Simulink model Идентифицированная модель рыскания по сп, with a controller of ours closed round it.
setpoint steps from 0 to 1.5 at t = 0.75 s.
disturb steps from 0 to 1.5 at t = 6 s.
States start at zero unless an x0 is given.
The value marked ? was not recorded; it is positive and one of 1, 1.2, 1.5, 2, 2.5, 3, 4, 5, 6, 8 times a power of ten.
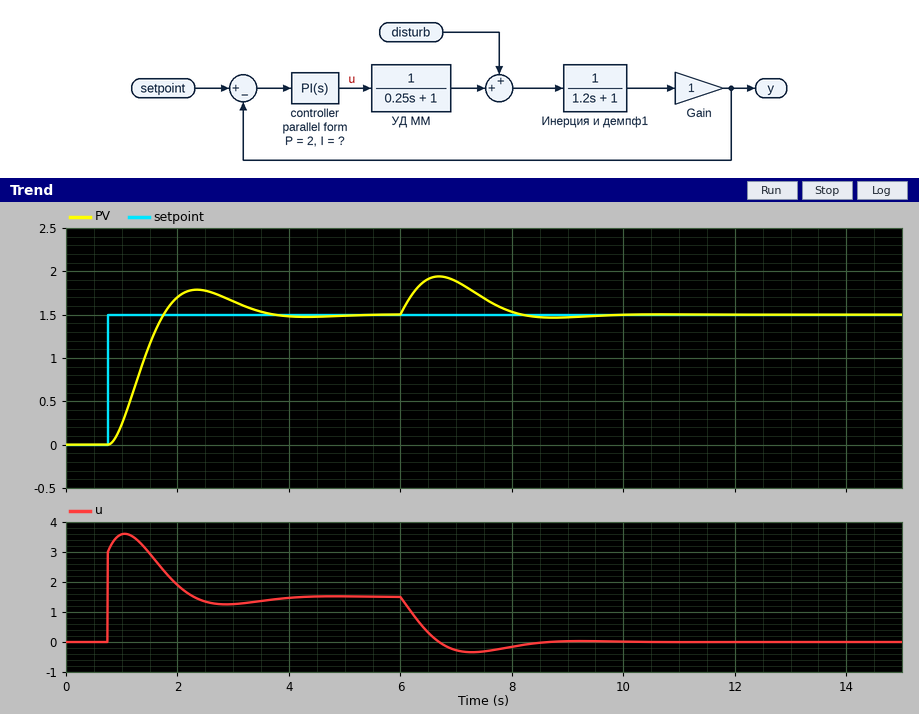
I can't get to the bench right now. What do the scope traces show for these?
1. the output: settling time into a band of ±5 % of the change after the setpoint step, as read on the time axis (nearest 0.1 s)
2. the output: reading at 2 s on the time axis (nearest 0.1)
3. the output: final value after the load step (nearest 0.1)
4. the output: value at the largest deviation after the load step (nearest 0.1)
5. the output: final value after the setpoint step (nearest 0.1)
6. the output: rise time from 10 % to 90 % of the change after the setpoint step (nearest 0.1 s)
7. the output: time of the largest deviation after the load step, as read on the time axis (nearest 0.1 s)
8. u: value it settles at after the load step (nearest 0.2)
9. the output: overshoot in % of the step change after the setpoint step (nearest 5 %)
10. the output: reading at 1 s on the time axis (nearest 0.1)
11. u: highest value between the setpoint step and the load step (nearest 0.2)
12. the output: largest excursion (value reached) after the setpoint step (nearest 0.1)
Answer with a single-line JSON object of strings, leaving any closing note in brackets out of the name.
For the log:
{"the output: settling time into a band of ±5 % of the change after the setpoint step, as read on the time axis": "3.3 s", "the output: reading at 2 s on the time axis": "1.7", "the output: final value after the load step": "1.5", "the output: value at the largest deviation after the load step": "1.9", "the output: final value after the setpoint step": "1.5", "the output: rise time from 10 % to 90 % of the change after the setpoint step": "0.7 s", "the output: time of the largest deviation after the load step, as read on the time axis": "6.7 s", "u: value it settles at after the load step": "0.0", "the output: overshoot in % of the step change after the setpoint step": "20 %", "the output: reading at 1 s on the time axis": "0.2", "u: highest value between the setpoint step and the load step": "3.6", "the output: largest excursion (value reached) after the setpoint step": "1.8"}
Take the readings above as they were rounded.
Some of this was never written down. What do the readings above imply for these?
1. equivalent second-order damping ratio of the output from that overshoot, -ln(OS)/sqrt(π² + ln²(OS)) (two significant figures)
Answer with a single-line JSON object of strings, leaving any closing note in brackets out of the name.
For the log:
{"equivalent second-order damping ratio of the output from that overshoot, -ln(OS)/sqrt(π² + ln²(OS))": "0.46"}
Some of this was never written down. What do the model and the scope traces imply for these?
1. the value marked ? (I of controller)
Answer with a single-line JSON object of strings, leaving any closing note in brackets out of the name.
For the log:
{"the value marked ?": "3"}
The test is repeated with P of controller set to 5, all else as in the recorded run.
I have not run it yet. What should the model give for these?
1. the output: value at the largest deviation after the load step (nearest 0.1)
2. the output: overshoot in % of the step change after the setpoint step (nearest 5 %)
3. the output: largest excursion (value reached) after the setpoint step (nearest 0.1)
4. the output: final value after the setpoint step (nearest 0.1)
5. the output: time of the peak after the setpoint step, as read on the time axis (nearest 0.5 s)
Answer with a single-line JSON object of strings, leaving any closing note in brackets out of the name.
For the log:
{"the output: value at the largest deviation after the load step": "1.8", "the output: overshoot in % of the step change after the setpoint step": "10 %", "the output: largest excursion (value reached) after the setpoint step": "1.7", "the output: final value after the setpoint step": "1.5", "the output: time of the peak after the setpoint step, as read on the time axis": "1.5 s"}
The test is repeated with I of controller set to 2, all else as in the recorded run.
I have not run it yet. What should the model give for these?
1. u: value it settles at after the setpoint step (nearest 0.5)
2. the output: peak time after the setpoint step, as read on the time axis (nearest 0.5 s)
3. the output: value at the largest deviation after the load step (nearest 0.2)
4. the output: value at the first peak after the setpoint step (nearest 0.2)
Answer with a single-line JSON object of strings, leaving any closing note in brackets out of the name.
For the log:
{"u: value it settles at after the setpoint step": "1.5", "the output: peak time after the setpoint step, as read on the time axis": "2.5 s", "the output: value at the largest deviation after the load step": "2.0", "the output: value at the first peak after the setpoint step": "1.6"}
